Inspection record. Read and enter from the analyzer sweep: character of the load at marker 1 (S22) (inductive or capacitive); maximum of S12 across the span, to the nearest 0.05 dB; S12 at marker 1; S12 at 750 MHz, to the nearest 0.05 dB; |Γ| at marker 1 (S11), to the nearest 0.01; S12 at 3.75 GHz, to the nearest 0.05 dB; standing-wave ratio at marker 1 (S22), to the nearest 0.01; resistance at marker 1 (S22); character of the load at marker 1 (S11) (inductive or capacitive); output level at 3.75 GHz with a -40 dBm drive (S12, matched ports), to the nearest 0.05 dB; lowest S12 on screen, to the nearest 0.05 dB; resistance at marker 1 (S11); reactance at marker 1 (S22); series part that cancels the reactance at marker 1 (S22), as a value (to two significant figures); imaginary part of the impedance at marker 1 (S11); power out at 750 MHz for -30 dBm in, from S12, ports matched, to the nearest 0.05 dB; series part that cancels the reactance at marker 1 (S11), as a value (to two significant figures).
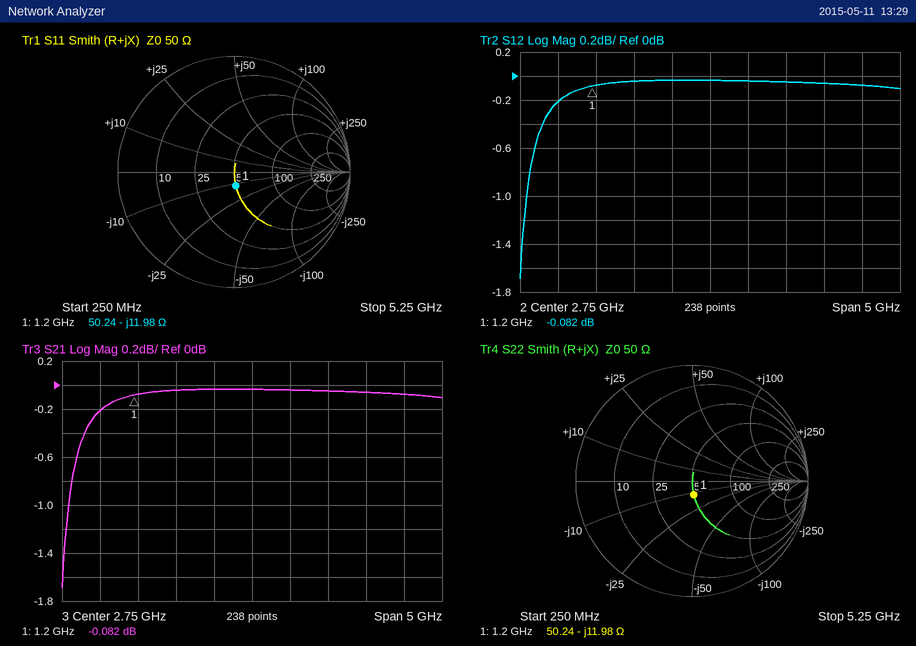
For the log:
capacitive
-0.05 dB
-0.082 dB
-0.20 dB
0.12
-0.05 dB
1.27
50.24 Ω
capacitive
-40.05 dBm
-1.70 dB
50.24 Ω
-11.98 Ω
1.6 nH
-11.98 Ω
-30.20 dBm
1.6 nH
